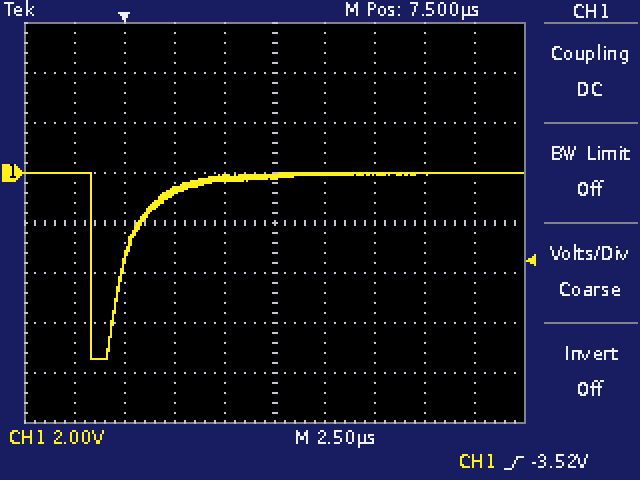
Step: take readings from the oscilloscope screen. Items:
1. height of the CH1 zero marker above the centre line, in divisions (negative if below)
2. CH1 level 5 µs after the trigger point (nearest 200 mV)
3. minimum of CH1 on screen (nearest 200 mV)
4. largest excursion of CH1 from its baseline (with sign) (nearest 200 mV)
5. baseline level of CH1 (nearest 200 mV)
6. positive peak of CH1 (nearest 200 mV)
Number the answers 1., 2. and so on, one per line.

1. +1.0 div
2. -200 mV
3. -7.4 V
4. -7.4 V
5. 0.0 V
6. 0.0 V
